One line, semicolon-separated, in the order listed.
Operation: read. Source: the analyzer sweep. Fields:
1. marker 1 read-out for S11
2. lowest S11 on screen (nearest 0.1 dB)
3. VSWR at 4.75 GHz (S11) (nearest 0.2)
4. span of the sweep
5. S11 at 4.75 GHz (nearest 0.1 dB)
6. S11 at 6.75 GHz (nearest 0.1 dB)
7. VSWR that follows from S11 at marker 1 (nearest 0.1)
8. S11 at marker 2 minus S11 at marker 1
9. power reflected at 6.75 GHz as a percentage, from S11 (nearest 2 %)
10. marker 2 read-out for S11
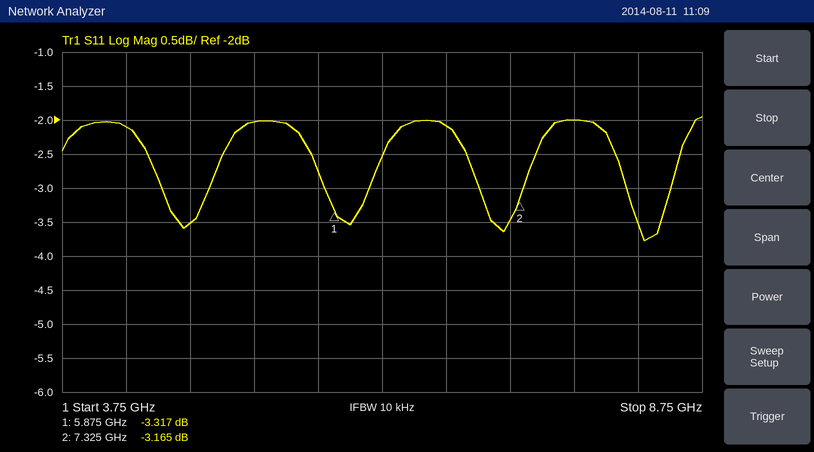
-3.317 dB; -3.8 dB; 5.0; 5 GHz; -3.5 dB; -2.1 dB; 5.3; 0.152 dB; 62 %; -3.165 dB
